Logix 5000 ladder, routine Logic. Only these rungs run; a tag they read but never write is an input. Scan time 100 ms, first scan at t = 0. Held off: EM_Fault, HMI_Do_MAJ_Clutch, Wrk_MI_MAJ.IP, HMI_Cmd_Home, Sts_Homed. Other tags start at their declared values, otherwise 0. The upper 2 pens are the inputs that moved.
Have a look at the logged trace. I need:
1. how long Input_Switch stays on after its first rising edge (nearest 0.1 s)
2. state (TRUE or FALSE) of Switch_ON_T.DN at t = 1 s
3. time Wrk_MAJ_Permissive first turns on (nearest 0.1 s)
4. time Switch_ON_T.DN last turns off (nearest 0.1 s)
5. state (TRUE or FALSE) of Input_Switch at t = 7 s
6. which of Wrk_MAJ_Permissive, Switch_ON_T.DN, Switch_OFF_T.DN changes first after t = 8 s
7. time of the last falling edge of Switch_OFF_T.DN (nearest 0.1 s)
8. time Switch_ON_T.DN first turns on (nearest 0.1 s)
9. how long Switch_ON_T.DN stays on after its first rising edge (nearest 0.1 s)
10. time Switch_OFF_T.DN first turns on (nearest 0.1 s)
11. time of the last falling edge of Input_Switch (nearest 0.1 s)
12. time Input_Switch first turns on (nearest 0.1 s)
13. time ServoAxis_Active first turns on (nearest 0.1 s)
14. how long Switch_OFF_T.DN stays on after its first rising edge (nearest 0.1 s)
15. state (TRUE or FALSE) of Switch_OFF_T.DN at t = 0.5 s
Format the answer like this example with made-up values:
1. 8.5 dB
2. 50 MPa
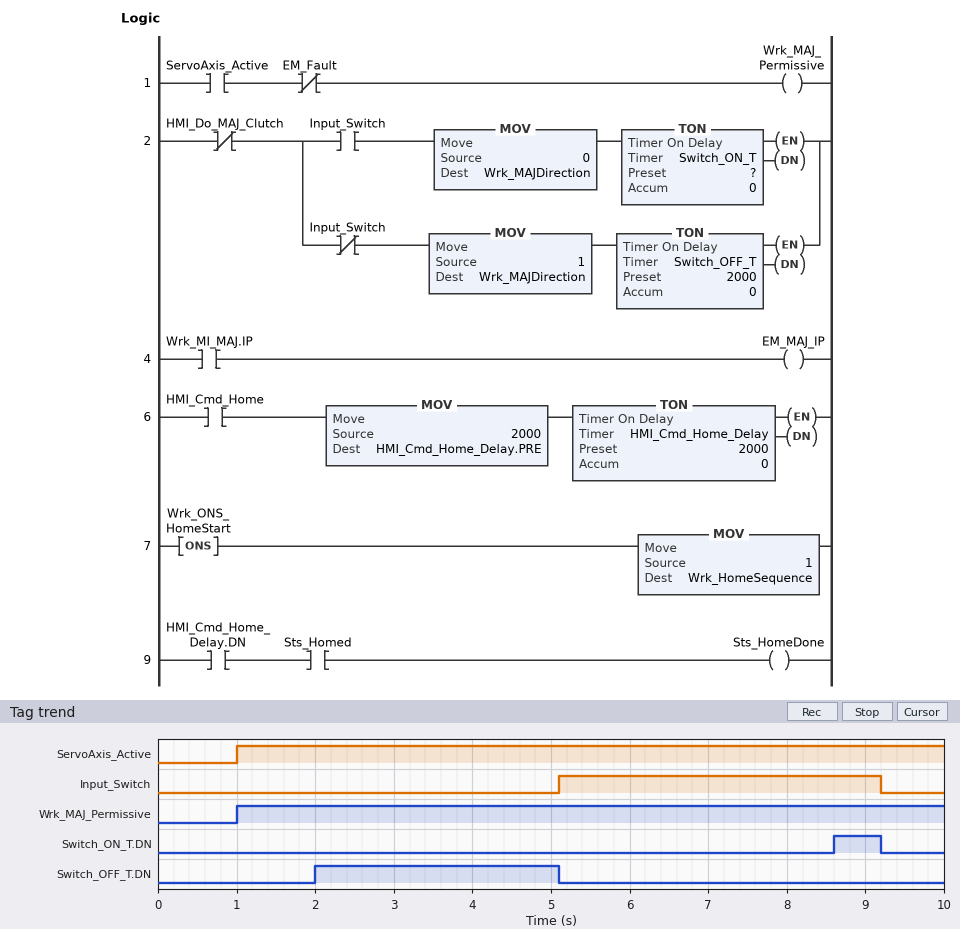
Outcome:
1. 4.1 s
2. FALSE
3. 1.0 s
4. 9.2 s
5. TRUE
6. Switch_ON_T.DN
7. 5.1 s
8. 8.6 s
9. 0.6 s
10. 2.0 s
11. 9.2 s
12. 5.1 s
13. 1.0 s
14. 3.1 s
15. FALSE
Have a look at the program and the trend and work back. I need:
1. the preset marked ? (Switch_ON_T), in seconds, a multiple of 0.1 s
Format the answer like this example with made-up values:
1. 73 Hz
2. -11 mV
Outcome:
1. 3.5 s
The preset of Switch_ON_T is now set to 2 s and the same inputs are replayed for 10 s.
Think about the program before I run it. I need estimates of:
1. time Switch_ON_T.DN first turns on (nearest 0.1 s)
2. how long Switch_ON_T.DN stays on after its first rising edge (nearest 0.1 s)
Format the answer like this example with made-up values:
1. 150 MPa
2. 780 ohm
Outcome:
1. 7.1 s
2. 2.1 s
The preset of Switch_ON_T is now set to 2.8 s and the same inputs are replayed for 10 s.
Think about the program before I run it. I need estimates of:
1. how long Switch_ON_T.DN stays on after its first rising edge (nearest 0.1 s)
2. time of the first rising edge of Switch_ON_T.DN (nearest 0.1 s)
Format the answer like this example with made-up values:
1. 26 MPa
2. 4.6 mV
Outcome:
1. 1.3 s
2. 7.9 s
